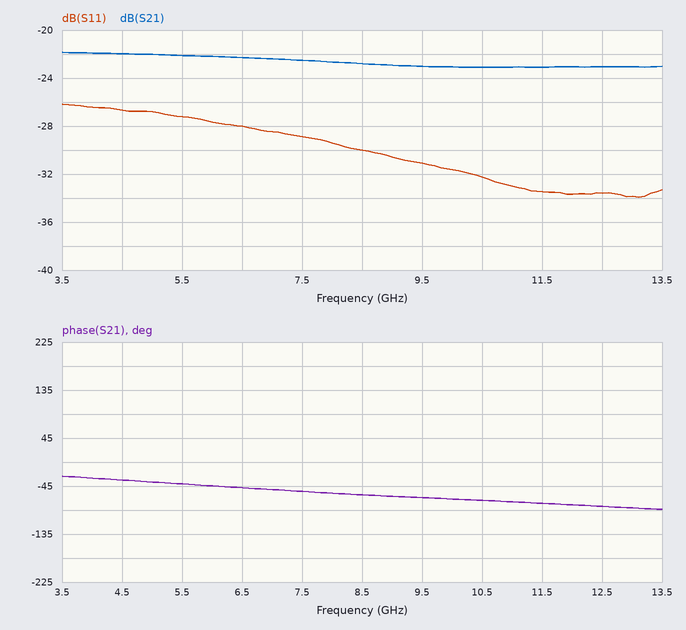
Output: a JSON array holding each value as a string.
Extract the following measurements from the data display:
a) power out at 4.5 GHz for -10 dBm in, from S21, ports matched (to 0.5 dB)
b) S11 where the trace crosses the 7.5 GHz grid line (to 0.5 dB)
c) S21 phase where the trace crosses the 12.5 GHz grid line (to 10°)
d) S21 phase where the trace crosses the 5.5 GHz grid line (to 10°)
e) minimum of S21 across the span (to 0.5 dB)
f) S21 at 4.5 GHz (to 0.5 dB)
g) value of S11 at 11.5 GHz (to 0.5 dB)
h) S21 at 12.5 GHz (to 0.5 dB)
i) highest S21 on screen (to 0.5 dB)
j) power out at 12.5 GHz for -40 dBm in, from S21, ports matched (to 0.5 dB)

["-32.0 dBm", "-29.0 dB", "-80°", "-40°", "-23.0 dB", "-22.0 dB", "-33.5 dB", "-23.0 dB", "-22.0 dB", "-63.0 dBm"]
